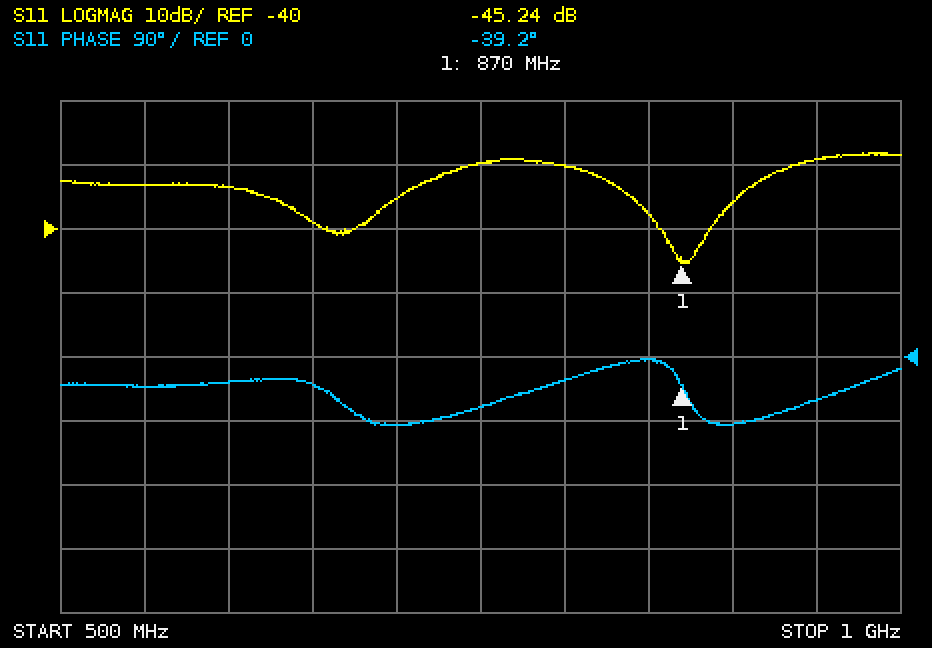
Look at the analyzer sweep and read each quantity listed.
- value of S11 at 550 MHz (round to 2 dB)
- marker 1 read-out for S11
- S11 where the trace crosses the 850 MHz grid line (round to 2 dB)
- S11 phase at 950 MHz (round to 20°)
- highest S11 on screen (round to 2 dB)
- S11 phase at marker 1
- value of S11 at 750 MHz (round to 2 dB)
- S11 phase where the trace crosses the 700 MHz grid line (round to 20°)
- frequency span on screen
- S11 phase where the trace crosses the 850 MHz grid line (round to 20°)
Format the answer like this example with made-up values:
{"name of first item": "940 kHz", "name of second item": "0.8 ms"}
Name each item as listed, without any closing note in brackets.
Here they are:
{"value of S11 at 550 MHz": "-34 dB", "marker 1 read-out for S11": "-45.24 dB", "S11 where the trace crosses the 850 MHz grid line": "-38 dB", "S11 phase at 950 MHz": "-60°", "highest S11 on screen": "-28 dB", "S11 phase at marker 1": "-39.2°", "value of S11 at 750 MHz": "-30 dB", "S11 phase where the trace crosses the 700 MHz grid line": "-100°", "frequency span on screen": "500 MHz", "S11 phase where the trace crosses the 850 MHz grid line": "0°"}
